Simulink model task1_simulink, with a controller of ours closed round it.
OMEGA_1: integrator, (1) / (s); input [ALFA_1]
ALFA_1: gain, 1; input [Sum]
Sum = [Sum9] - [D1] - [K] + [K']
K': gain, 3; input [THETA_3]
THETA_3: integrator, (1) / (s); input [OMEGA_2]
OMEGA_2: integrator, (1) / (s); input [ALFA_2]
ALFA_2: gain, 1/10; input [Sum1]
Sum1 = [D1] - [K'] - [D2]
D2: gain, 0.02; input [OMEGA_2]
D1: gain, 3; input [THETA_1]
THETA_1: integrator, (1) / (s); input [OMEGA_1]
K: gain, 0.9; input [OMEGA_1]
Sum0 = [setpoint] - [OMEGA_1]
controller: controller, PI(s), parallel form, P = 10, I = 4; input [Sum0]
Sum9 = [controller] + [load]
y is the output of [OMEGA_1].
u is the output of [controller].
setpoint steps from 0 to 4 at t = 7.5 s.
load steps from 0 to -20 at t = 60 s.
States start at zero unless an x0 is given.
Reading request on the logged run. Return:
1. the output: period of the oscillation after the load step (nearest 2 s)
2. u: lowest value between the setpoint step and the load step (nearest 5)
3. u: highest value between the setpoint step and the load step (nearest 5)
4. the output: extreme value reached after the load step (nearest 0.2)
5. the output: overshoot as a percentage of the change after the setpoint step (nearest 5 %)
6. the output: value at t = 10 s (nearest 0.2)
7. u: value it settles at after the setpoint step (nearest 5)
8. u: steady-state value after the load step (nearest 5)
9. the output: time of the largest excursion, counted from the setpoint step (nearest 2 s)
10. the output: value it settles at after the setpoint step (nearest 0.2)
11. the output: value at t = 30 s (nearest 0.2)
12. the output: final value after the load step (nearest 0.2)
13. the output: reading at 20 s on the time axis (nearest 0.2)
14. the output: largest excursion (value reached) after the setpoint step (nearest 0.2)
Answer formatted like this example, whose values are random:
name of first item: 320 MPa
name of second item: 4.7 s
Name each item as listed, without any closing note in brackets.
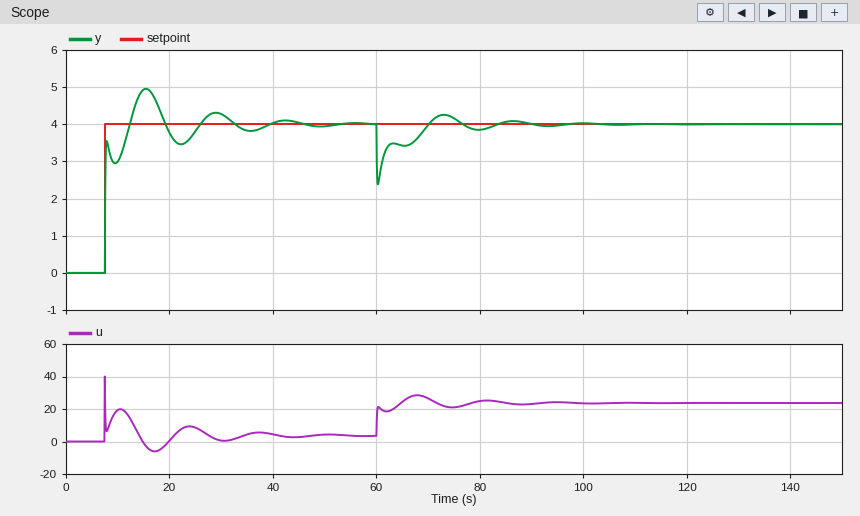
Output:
the output: period of the oscillation after the load step: 20 s
u: lowest value between the setpoint step and the load step: -5
u: highest value between the setpoint step and the load step: 40
the output: extreme value reached after the load step: 2.4
the output: overshoot as a percentage of the change after the setpoint step: 25 %
the output: value at t = 10 s: 3.0
u: value it settles at after the setpoint step: 5
u: steady-state value after the load step: 25
the output: time of the largest excursion, counted from the setpoint step: 8 s
the output: value it settles at after the setpoint step: 4.0
the output: value at t = 30 s: 4.2
the output: final value after the load step: 4.0
the output: reading at 20 s on the time axis: 3.8
the output: largest excursion (value reached) after the setpoint step: 5.0
